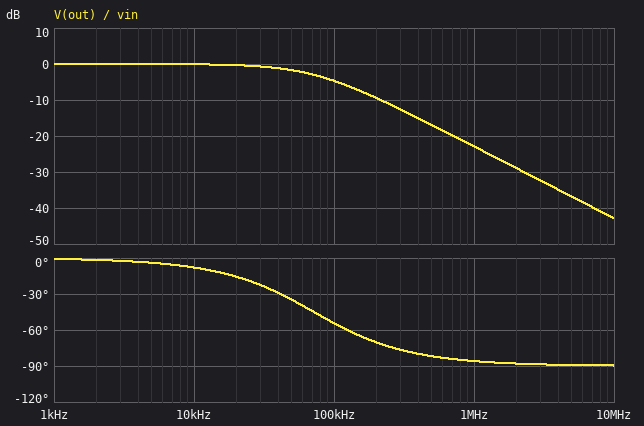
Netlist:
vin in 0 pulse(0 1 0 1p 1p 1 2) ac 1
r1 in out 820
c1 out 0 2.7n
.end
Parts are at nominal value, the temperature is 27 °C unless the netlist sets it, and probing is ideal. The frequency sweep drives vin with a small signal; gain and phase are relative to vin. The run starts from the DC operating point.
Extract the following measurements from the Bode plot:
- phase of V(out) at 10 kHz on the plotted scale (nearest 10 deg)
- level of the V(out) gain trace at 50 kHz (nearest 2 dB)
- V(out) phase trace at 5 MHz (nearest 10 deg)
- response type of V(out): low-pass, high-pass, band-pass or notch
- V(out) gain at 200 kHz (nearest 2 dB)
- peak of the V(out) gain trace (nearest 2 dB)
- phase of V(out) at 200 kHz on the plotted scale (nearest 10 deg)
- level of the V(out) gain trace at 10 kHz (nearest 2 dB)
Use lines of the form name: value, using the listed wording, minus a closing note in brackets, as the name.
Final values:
phase of V(out) at 10 kHz on the plotted scale: -10 deg
level of the V(out) gain trace at 50 kHz: -2 dB
V(out) phase trace at 5 MHz: -90 deg
response type of V(out): low-pass, high-pass, band-pass or notch: low-pass
V(out) gain at 200 kHz: -10 dB
peak of the V(out) gain trace: 0 dB
phase of V(out) at 200 kHz on the plotted scale: -70 deg
level of the V(out) gain trace at 10 kHz: 0 dB
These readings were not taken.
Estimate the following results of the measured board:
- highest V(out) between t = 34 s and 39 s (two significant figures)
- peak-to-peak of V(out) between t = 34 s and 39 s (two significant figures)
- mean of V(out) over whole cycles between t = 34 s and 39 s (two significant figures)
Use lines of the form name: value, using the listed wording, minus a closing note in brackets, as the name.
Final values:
highest V(out) between t = 34 s and 39 s: 1.0 V
peak-to-peak of V(out) between t = 34 s and 39 s: 1.0 V
mean of V(out) over whole cycles between t = 34 s and 39 s: 500 mV
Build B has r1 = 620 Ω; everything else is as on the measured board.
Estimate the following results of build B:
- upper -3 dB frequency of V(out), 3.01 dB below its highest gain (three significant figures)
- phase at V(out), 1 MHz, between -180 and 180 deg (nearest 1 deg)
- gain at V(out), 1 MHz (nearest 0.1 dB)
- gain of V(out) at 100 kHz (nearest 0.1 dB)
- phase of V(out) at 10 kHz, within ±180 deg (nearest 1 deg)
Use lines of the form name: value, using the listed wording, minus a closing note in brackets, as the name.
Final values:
upper -3 dB frequency of V(out), 3.01 dB below its highest gain: 95.1 kHz
phase at V(out), 1 MHz, between -180 and 180 deg: -85 deg
gain at V(out), 1 MHz: -20.5 dB
gain of V(out) at 100 kHz: -3.2 dB
phase of V(out) at 10 kHz, within ±180 deg: -6 deg
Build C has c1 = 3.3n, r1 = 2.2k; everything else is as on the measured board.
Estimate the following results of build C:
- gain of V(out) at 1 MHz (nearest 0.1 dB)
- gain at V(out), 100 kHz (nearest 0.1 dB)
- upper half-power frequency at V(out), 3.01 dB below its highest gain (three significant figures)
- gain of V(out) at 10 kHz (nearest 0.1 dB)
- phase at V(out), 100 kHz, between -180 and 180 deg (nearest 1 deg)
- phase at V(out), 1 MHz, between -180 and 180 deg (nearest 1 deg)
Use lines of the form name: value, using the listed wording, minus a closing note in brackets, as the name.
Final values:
gain of V(out) at 1 MHz: -33.2 dB
gain at V(out), 100 kHz: -13.4 dB
upper half-power frequency at V(out), 3.01 dB below its highest gain: 21.9 kHz
gain of V(out) at 10 kHz: -0.8 dB
phase at V(out), 100 kHz, between -180 and 180 deg: -78 deg
phase at V(out), 1 MHz, between -180 and 180 deg: -89 deg
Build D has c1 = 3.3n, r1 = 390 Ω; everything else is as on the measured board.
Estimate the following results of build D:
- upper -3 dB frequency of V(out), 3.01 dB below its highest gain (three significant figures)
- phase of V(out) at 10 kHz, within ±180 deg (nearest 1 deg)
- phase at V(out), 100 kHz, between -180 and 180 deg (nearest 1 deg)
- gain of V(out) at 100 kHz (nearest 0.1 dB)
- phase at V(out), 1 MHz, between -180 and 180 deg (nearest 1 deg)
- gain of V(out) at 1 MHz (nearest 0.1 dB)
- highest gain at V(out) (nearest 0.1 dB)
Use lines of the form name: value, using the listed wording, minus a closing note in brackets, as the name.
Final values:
upper -3 dB frequency of V(out), 3.01 dB below its highest gain: 124 kHz
phase of V(out) at 10 kHz, within ±180 deg: -5 deg
phase at V(out), 100 kHz, between -180 and 180 deg: -39 deg
gain of V(out) at 100 kHz: -2.2 dB
phase at V(out), 1 MHz, between -180 and 180 deg: -83 deg
gain of V(out) at 1 MHz: -18.2 dB
highest gain at V(out): 0 dB
